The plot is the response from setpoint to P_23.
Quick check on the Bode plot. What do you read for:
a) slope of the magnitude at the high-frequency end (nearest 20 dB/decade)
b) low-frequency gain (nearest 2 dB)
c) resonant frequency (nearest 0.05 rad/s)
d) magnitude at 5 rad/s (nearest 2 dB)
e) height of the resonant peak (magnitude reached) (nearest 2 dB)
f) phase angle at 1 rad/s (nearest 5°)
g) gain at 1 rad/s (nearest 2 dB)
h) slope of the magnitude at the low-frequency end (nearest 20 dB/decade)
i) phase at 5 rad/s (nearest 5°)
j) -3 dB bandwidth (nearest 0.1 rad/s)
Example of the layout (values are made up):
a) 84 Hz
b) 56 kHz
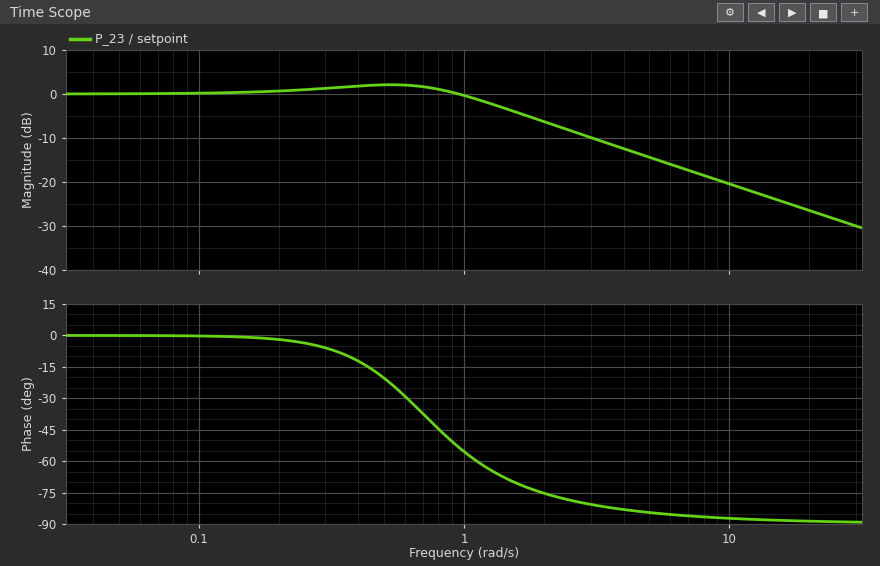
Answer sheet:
a) -20 dB/decade
b) 0 dB
c) 0.50 rad/s
d) -14 dB
e) 2 dB
f) -55°
g) 0 dB
h) 0 dB/decade
i) -85°
j) 1.4 rad/s
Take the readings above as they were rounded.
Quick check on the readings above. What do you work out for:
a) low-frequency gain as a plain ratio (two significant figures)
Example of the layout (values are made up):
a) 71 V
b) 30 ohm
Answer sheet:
a) 1.0
